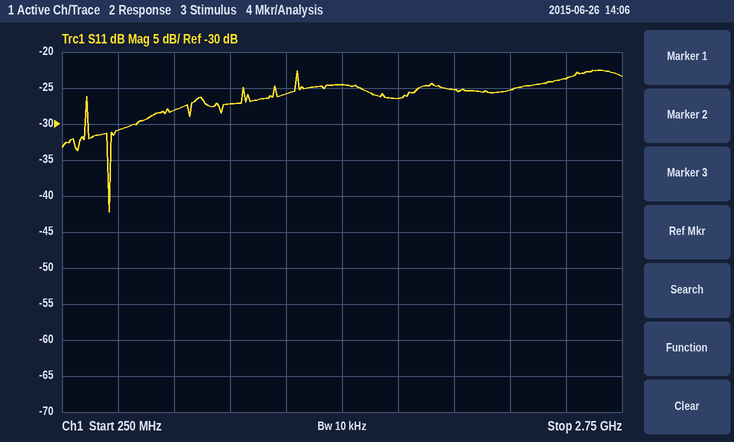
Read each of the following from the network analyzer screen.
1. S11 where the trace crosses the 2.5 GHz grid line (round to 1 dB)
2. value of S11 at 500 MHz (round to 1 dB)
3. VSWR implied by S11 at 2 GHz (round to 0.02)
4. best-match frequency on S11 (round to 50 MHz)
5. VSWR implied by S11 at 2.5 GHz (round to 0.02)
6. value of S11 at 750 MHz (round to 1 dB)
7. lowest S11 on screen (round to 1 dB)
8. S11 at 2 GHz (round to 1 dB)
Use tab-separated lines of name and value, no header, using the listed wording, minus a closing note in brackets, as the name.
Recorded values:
S11 where the trace crosses the 2.5 GHz grid line	-24 dB
value of S11 at 500 MHz	-31 dB
VSWR implied by S11 at 2 GHz	1.12
best-match frequency on S11	450 MHz
VSWR implied by S11 at 2.5 GHz	1.14
value of S11 at 750 MHz	-28 dB
lowest S11 on screen	-42 dB
S11 at 2 GHz	-25 dB
